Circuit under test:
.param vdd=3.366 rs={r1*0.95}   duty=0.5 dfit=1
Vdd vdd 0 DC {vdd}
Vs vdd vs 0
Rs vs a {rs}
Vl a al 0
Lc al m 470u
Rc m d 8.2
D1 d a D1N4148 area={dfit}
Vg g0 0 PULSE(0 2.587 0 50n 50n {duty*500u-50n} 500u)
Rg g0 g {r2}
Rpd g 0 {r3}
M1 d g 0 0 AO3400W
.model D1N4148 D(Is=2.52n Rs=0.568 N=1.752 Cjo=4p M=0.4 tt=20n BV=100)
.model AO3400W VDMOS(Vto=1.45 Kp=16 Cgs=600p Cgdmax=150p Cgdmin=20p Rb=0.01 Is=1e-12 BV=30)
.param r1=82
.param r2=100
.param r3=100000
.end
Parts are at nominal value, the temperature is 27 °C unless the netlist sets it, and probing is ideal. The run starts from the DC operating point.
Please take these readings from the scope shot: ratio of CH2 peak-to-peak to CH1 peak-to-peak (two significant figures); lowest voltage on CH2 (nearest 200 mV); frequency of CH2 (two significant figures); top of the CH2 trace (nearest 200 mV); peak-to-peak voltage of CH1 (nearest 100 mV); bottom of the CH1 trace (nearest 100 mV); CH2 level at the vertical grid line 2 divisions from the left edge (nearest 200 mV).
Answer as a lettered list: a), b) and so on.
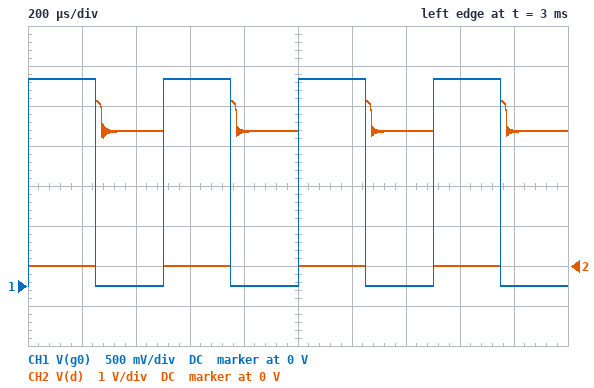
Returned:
a) 1.6
b) 0 V
c) 2.0 kHz
d) 4.2 V
e) 2.6 V
f) 0 V
g) 3.4 V
